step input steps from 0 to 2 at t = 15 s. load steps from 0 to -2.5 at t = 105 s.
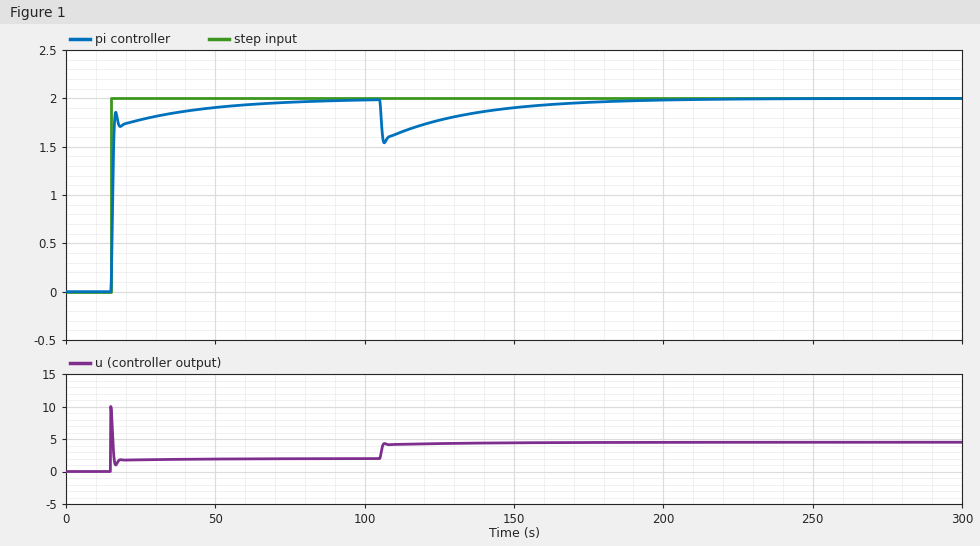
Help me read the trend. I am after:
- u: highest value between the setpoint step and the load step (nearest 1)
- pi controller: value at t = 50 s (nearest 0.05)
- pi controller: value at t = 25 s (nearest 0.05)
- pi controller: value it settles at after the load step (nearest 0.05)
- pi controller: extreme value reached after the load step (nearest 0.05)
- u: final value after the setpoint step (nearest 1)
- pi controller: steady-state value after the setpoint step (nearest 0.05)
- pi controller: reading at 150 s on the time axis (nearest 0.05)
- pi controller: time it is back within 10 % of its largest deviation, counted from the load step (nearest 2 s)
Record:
10
1.90
1.80
2.00
1.55
2
2.00
1.90
68 s
